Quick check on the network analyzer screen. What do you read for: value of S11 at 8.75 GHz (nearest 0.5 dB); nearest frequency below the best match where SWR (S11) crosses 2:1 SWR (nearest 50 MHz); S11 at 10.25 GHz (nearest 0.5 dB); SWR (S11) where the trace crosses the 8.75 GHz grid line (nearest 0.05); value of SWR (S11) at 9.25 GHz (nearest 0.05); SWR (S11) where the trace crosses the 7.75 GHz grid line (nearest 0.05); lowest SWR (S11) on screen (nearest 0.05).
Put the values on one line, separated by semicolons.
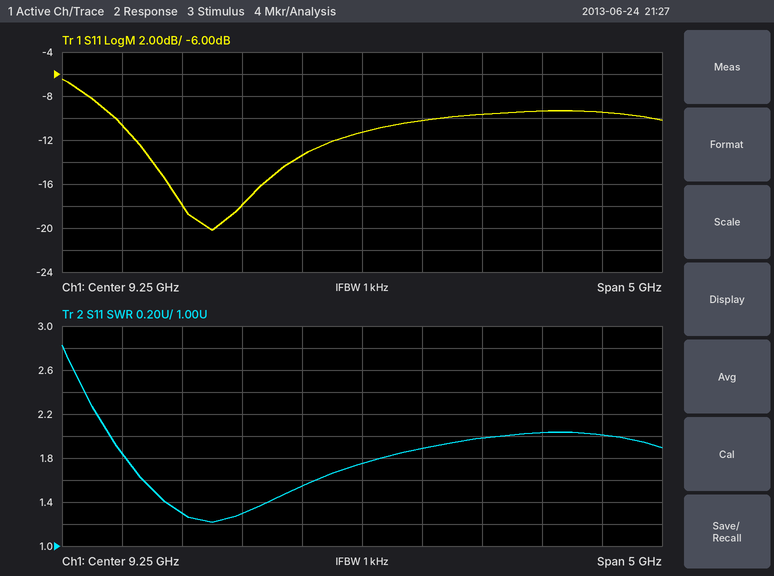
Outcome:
-13.5 dB; 7.15 GHz; -9.5 dB; 1.55; 1.75; 1.30; 1.20
